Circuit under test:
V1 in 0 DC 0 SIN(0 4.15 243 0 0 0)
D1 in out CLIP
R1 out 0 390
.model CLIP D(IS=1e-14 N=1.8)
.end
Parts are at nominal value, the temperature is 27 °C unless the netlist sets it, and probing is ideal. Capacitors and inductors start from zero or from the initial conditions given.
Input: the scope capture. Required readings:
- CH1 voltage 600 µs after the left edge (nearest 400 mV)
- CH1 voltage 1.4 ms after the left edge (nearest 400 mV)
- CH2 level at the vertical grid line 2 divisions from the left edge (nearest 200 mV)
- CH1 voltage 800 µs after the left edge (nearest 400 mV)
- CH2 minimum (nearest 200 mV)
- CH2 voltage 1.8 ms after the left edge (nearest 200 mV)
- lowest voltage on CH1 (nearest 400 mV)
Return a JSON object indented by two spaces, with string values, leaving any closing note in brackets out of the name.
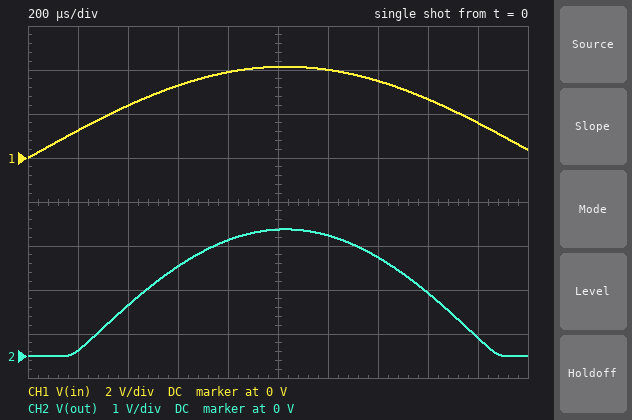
{
  "CH1 voltage 600 µs after the left edge": "3.2 V",
  "CH1 voltage 1.4 ms after the left edge": "3.6 V",
  "CH2 level at the vertical grid line 2 divisions from the left edge": "1.2 V",
  "CH1 voltage 800 µs after the left edge": "4.0 V",
  "CH2 minimum": "0 V",
  "CH2 voltage 1.8 ms after the left edge": "400 mV",
  "lowest voltage on CH1": "0 V"
}
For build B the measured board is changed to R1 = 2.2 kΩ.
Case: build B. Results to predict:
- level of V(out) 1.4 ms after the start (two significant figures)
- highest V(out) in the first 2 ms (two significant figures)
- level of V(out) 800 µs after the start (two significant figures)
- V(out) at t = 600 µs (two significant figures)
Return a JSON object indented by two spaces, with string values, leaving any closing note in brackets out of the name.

{
  "level of V(out) 1.4 ms after the start": "2.3 V",
  "highest V(out) in the first 2 ms": "3.0 V",
  "level of V(out) 800 µs after the start": "2.7 V",
  "V(out) at t = 600 µs": "2.1 V"
}
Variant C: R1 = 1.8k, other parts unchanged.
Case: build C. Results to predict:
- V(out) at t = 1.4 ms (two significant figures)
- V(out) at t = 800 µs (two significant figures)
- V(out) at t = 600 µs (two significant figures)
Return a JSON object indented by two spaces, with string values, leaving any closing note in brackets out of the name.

{
  "V(out) at t = 1.4 ms": "2.3 V",
  "V(out) at t = 800 µs": "2.7 V",
  "V(out) at t = 600 µs": "2.1 V"
}
